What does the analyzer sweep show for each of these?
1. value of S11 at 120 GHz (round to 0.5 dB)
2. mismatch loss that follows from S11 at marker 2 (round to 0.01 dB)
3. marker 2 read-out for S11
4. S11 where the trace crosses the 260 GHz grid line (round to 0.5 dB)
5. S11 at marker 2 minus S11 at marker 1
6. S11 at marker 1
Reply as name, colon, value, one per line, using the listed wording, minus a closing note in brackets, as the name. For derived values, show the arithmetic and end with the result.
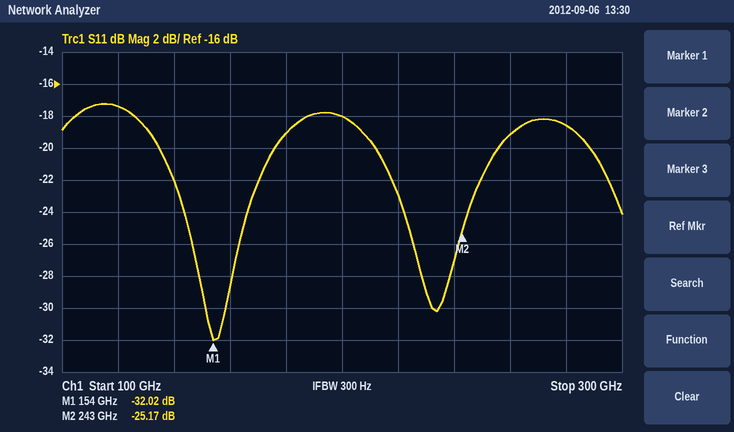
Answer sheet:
value of S11 at 120 GHz: -17.5 dB
mismatch loss that follows from S11 at marker 2: −10 log10(1 − 10^(-25.17/10)) ≈ 0.01 dB
marker 2 read-out for S11: -25.17 dB
S11 where the trace crosses the 260 GHz grid line: -19.0 dB
S11 at marker 2 minus S11 at marker 1: -25.17 − (-32.02) = 6.85 dB
S11 at marker 1: -32.02 dB
